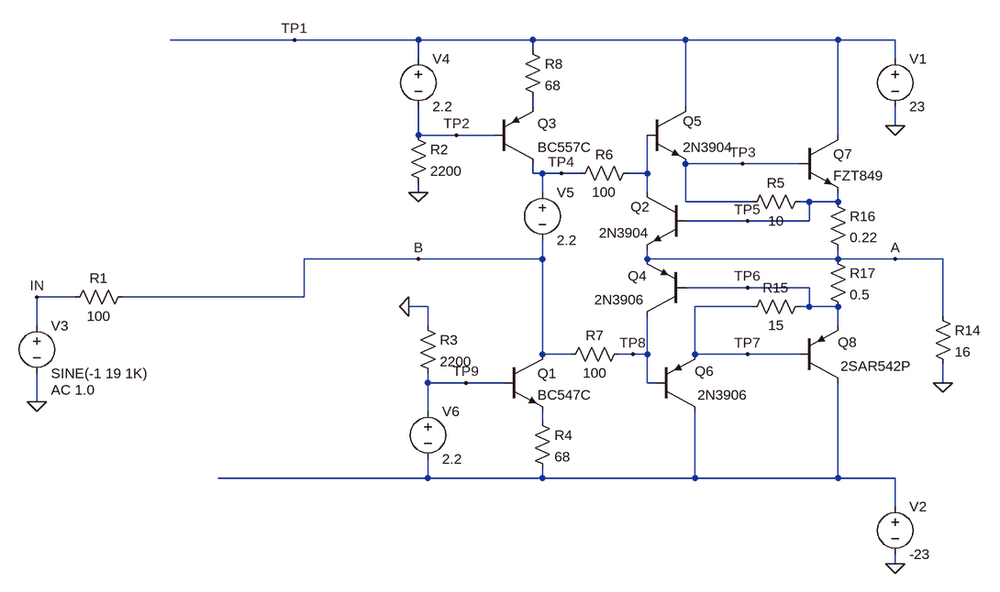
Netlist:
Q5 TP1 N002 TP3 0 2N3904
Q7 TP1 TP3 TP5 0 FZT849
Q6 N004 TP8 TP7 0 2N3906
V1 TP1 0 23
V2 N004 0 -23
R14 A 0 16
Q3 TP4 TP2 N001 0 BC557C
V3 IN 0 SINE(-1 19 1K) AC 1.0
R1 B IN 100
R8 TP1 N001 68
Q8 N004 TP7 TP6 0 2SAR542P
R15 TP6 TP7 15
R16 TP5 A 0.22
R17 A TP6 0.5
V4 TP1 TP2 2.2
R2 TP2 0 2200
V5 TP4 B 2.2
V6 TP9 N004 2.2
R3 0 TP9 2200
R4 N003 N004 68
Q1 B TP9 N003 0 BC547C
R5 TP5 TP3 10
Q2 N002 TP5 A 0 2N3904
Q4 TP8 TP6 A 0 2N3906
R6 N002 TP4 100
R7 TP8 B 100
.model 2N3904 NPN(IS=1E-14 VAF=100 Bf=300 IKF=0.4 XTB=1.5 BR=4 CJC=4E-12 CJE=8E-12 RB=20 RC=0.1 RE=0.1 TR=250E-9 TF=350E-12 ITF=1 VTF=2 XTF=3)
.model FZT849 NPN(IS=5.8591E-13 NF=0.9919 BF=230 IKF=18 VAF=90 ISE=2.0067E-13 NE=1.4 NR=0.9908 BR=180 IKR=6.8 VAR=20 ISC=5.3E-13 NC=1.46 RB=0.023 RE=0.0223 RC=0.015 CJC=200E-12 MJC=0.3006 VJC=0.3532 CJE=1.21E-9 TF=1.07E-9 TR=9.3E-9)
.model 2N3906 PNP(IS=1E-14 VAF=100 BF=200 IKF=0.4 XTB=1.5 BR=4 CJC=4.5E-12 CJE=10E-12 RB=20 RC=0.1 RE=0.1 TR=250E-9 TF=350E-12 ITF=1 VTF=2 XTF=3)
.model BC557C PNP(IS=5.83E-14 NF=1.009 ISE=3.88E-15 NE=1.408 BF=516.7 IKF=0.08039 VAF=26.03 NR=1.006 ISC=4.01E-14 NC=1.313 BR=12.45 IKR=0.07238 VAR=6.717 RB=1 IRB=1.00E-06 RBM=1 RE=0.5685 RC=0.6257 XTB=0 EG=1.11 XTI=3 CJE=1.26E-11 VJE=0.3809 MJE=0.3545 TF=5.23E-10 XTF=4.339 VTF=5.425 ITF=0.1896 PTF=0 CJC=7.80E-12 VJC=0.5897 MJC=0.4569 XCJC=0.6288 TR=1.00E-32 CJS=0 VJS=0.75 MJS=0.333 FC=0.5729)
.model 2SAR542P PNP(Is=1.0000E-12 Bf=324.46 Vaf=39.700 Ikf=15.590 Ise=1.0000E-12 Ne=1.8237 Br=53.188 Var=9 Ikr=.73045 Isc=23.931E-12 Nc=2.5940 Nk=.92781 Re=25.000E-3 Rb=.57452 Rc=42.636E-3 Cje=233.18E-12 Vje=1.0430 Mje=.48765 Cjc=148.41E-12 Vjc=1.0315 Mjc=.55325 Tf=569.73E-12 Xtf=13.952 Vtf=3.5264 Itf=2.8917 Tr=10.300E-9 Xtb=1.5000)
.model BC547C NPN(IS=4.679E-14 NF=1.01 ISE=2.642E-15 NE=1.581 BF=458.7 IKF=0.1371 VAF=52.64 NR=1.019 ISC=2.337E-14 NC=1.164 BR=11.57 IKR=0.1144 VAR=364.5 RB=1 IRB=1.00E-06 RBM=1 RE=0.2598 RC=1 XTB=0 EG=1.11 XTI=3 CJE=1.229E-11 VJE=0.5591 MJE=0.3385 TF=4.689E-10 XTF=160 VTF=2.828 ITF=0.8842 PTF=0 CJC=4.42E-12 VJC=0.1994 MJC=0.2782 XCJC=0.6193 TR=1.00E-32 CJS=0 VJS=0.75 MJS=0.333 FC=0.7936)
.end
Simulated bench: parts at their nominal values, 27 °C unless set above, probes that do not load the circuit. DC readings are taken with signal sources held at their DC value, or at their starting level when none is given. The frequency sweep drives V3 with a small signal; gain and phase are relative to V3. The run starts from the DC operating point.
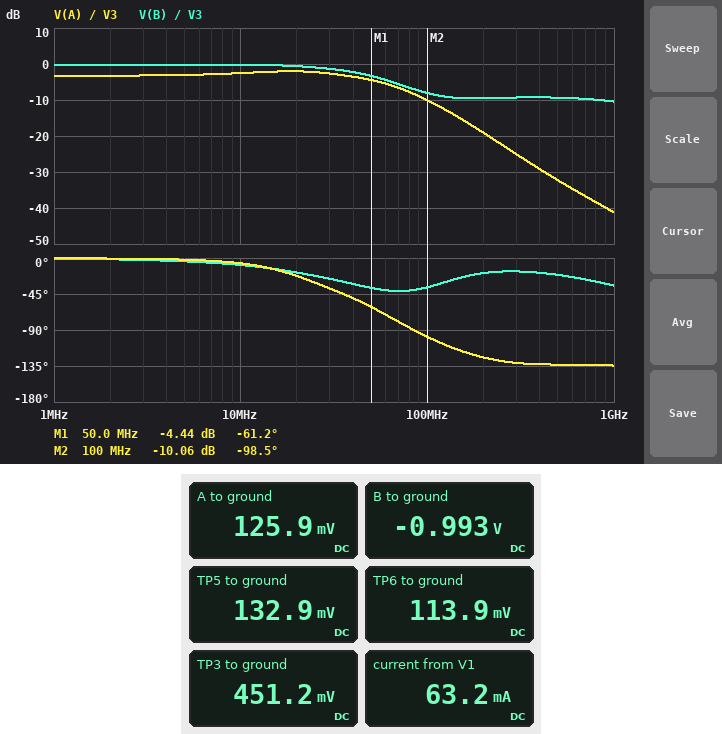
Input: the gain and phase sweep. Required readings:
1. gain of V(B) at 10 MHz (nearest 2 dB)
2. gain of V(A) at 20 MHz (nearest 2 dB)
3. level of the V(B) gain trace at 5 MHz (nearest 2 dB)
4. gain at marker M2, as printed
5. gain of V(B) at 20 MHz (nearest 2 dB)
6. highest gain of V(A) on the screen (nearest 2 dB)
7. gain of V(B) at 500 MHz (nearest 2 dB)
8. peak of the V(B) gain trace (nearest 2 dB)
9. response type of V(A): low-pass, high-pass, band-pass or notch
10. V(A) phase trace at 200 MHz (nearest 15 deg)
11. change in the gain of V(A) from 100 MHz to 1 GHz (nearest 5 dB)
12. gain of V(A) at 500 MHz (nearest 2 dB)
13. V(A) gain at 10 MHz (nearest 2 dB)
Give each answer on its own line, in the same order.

0 dB
-2 dB
0 dB
-10.06 dB
0 dB
-2 dB
-10 dB
0 dB
low-pass
-120 deg
-30 dB
-32 dB
-2 dB
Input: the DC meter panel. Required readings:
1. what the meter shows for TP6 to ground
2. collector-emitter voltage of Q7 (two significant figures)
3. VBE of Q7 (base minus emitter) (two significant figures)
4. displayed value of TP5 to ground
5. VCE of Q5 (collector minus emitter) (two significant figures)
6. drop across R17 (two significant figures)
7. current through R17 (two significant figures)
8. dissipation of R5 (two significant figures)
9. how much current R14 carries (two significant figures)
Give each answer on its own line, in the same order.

113.9 mV
23 V
320 mV
132.9 mV
23 V
12 mV
24 mA
10 mW
7.9 mA
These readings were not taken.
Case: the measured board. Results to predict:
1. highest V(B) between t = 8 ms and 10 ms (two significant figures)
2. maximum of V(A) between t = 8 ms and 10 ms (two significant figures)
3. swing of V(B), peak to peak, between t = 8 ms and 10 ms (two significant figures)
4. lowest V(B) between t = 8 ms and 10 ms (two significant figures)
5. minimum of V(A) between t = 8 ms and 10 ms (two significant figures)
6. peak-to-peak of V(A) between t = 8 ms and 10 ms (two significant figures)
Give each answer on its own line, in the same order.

18 V
18 V
38 V
-20 V
-18 V
36 V
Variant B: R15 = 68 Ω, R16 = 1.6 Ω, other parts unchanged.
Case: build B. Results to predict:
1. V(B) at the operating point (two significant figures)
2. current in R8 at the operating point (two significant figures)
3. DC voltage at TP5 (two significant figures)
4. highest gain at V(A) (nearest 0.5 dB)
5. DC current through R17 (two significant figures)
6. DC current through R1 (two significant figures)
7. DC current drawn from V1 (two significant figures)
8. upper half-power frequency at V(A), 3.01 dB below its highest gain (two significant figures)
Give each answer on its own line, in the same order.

-1.0 V
22 mA
250 mV
-2.5 dB
7.8 mA
25 µA
53 mA
58 MHz
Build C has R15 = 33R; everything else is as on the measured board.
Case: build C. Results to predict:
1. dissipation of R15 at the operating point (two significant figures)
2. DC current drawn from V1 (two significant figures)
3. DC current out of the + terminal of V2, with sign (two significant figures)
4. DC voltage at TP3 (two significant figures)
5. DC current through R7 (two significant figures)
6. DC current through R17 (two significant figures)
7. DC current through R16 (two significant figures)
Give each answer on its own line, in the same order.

6.3 mW
57 mA
-45 mA
460 mV
58 µA
14 mA
26 mA
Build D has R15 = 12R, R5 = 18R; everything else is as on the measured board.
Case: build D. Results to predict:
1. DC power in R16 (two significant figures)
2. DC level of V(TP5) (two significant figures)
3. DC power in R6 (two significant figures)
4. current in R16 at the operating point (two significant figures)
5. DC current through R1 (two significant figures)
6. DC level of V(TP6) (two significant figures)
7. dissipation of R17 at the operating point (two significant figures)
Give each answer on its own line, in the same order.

130 µW
34 mV
470 nW
24 mA
81 µA
18 mV
240 µW
